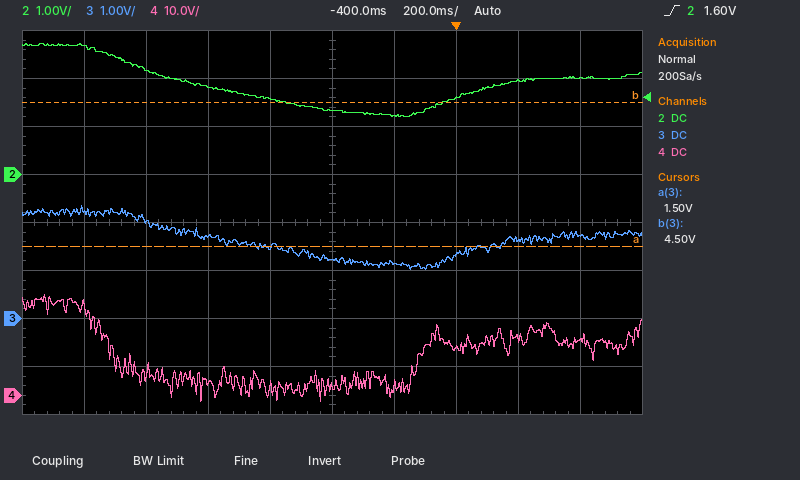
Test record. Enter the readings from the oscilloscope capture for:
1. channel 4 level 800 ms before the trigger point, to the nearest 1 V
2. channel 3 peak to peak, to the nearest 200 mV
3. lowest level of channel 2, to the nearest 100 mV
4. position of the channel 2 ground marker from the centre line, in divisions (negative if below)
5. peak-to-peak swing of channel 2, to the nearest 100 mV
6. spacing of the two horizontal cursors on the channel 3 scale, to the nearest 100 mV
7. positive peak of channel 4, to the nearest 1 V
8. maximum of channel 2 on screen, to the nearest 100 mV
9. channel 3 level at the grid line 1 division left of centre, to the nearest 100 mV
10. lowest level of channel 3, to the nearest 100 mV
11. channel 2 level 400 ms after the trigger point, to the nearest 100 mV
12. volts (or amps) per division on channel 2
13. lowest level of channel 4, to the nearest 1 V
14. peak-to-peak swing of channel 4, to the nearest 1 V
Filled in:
3 V
1.4 V
1.2 V
+1.0 div
1.5 V
3.0 V
21 V
2.7 V
1.5 V
1.0 V
2.0 V
1 V
-1 V
22 V
